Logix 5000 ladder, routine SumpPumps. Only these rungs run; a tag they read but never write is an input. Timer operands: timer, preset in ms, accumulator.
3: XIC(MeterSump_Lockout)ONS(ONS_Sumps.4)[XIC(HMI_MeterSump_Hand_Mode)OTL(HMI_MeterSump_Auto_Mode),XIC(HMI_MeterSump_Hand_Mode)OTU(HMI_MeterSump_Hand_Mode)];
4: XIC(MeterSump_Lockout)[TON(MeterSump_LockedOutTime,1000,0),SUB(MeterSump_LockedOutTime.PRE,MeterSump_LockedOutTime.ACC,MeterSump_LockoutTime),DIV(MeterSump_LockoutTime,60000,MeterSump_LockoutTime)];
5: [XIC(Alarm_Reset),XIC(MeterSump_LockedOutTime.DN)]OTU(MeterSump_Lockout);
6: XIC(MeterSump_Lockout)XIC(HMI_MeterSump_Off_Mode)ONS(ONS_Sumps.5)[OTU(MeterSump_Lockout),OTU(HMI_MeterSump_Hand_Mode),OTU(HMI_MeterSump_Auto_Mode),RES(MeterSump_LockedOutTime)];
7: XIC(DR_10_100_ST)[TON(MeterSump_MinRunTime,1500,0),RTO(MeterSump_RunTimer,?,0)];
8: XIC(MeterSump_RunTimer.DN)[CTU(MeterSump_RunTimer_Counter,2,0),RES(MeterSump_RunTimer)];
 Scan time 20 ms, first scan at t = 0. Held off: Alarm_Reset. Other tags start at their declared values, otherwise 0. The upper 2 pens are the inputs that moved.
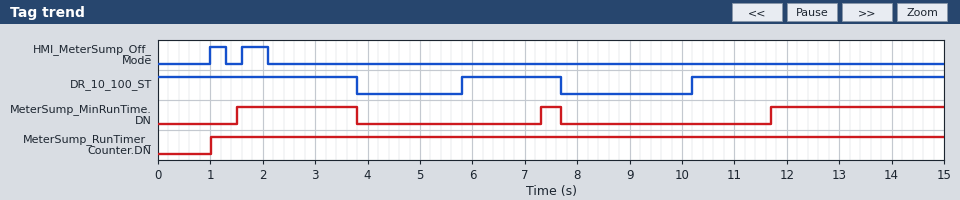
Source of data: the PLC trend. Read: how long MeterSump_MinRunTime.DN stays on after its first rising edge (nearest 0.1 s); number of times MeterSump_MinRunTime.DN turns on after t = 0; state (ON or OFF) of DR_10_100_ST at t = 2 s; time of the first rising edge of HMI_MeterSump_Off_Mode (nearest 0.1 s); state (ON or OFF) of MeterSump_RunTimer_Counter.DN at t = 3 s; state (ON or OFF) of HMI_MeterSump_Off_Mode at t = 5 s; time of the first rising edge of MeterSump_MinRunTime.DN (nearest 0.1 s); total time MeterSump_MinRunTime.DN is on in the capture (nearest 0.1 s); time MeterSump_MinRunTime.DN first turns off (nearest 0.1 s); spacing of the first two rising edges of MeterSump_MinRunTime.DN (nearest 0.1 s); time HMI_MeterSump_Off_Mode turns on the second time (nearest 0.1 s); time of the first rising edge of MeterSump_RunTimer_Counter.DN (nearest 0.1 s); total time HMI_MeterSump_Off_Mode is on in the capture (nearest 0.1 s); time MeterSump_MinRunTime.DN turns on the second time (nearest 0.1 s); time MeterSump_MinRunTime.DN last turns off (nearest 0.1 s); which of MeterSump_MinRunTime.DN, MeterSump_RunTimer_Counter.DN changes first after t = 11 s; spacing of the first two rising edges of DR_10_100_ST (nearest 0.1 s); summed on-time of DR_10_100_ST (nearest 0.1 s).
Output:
2.3 s
3
ON
1.0 s
ON
OFF
1.5 s
6.0 s
3.8 s
5.8 s
1.6 s
1.0 s
0.8 s
7.3 s
7.7 s
MeterSump_MinRunTime.DN
4.4 s
10.5 s
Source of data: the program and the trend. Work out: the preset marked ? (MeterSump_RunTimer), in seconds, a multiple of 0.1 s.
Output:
0.5 s
